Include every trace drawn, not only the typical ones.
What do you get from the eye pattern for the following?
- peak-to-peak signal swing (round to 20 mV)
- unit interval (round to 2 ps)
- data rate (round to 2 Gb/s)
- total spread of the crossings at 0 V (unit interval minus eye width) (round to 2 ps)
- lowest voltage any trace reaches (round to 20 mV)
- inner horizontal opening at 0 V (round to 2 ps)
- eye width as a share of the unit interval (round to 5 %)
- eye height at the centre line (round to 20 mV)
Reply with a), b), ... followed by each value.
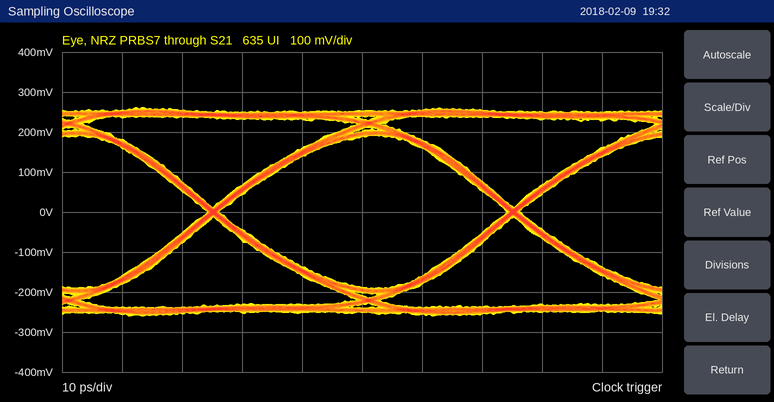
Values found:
a) 520 mV
b) 50 ps
c) 20 Gb/s
d) 2 ps
e) -260 mV
f) 48 ps
g) 95 %
h) 380 mV
